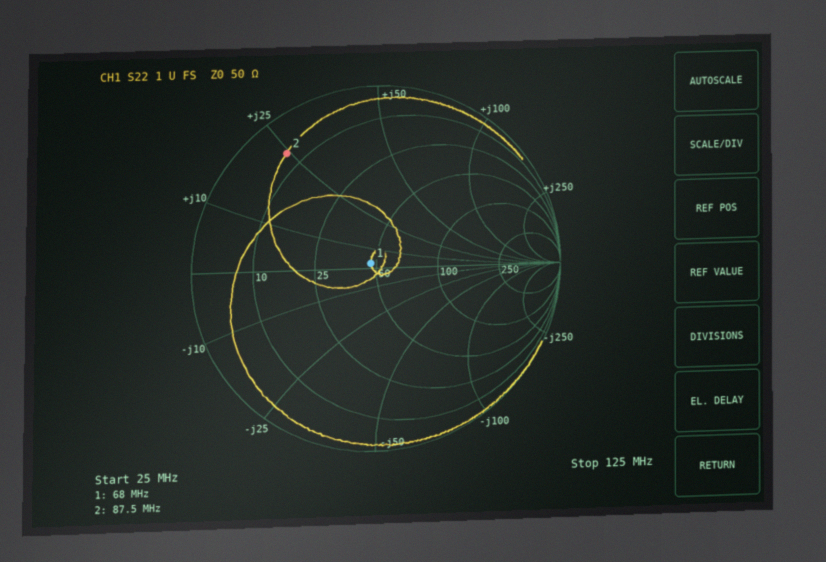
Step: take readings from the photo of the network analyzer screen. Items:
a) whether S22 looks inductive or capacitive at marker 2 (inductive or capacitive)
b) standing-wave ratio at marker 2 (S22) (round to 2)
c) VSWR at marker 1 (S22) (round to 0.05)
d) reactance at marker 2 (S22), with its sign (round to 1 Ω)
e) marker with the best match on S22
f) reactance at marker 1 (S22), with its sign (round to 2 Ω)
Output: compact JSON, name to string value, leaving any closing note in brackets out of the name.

{"whether S22 looks inductive or capacitive at marker 2": "inductive", "standing-wave ratio at marker 2 (S22)": "10", "VSWR at marker 1 (S22)": "1.10", "reactance at marker 2 (S22), with its sign": "+24 Ω", "marker with the best match on S22": "marker 1", "reactance at marker 1 (S22), with its sign": "+2 Ω"}
